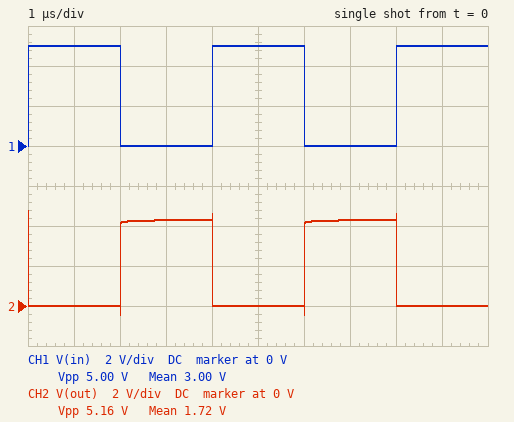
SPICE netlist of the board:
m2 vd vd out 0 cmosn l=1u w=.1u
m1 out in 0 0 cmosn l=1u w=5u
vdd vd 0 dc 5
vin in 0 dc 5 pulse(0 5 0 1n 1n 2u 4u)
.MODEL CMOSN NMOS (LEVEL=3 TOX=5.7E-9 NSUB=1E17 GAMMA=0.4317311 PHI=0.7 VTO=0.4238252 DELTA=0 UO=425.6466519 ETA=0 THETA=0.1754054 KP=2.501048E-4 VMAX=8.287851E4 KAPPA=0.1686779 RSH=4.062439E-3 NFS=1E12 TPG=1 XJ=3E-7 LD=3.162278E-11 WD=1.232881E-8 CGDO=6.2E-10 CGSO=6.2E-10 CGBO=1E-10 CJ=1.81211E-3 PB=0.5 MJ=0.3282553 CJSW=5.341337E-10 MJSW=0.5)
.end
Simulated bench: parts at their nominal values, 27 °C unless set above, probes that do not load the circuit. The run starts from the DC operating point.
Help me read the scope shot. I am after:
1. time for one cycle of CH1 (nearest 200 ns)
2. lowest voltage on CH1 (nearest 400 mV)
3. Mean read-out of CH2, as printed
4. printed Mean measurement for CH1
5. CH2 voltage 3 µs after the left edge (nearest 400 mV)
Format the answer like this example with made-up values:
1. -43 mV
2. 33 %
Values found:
1. 4.0 µs
2. 0 V
3. 1.72 V
4. 3.00 V
5. 4.4 V
